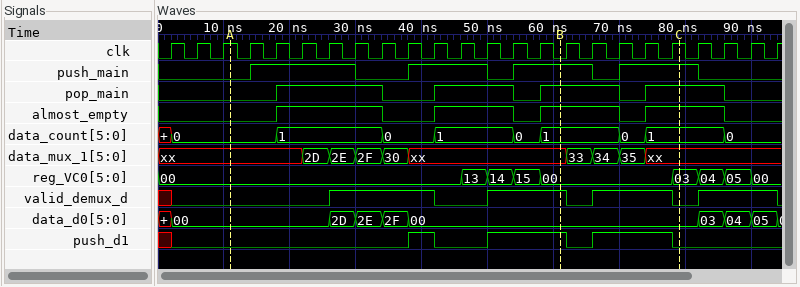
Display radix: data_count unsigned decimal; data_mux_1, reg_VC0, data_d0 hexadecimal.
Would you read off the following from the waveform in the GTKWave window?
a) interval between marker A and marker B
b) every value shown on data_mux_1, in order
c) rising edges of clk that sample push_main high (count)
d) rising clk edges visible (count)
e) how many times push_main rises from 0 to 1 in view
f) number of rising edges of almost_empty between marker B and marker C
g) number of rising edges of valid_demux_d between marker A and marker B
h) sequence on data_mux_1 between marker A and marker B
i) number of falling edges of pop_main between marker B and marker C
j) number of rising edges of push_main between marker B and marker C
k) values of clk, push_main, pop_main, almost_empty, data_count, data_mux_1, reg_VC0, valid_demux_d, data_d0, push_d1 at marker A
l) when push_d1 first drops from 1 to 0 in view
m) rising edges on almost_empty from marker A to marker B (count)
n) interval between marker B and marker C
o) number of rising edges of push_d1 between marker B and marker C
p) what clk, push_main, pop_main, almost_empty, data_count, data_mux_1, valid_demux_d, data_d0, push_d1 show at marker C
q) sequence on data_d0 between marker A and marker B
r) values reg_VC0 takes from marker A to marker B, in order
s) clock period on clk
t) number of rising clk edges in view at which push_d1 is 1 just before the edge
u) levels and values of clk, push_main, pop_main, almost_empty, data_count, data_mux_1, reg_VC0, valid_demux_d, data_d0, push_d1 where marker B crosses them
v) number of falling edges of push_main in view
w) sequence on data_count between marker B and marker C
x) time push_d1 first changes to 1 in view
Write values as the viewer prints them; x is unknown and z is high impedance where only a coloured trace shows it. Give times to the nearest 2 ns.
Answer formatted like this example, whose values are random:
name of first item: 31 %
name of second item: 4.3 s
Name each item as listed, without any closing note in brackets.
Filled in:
interval between marker A and marker B: 50 ns
every value shown on data_mux_1, in order: xx, 2D, 2E, 2F, 30, xx, 33, 34, 35, xx
rising edges of clk that sample push_main high: 13
rising clk edges visible: 24
how many times push_main rises from 0 to 1 in view: 4
number of rising edges of almost_empty between marker B and marker C: 1
number of rising edges of valid_demux_d between marker A and marker B: 2
sequence on data_mux_1 between marker A and marker B: xx, 2D, 2E, 2F, 30, xx
number of falling edges of pop_main between marker B and marker C: 1
number of rising edges of push_main between marker B and marker C: 1
values of clk, push_main, pop_main, almost_empty, data_count, data_mux_1, reg_VC0, valid_demux_d, data_d0, push_d1 at marker A: clk=1, push_main=0, pop_main=0, almost_empty=0, data_count=0, data_mux_1=xx, reg_VC0=00, valid_demux_d=0, data_d0=00, push_d1=0
when push_d1 first drops from 1 to 0 in view: 42 ns
rising edges on almost_empty from marker A to marker B: 3
interval between marker B and marker C: 18 ns
number of rising edges of push_d1 between marker B and marker C: 1
what clk, push_main, pop_main, almost_empty, data_count, data_mux_1, valid_demux_d, data_d0, push_d1 show at marker C: clk=1, push_main=1, pop_main=1, almost_empty=1, data_count=1, data_mux_1=xx, valid_demux_d=0, data_d0=00, push_d1=0
sequence on data_d0 between marker A and marker B: 00, 2D, 2E, 2F, 00
values reg_VC0 takes from marker A to marker B, in order: 00, 13, 14, 15, 00
clock period on clk: 4 ns
number of rising clk edges in view at which push_d1 is 1 just before the edge: 7
levels and values of clk, push_main, pop_main, almost_empty, data_count, data_mux_1, reg_VC0, valid_demux_d, data_d0, push_d1 where marker B crosses them: clk=0, push_main=1, pop_main=1, almost_empty=1, data_count=1, data_mux_1=xx, reg_VC0=00, valid_demux_d=1, data_d0=00, push_d1=1
number of falling edges of push_main in view: 4
sequence on data_count between marker B and marker C: 1, 0, 1
time push_d1 first changes to 1 in view: 38 ns
